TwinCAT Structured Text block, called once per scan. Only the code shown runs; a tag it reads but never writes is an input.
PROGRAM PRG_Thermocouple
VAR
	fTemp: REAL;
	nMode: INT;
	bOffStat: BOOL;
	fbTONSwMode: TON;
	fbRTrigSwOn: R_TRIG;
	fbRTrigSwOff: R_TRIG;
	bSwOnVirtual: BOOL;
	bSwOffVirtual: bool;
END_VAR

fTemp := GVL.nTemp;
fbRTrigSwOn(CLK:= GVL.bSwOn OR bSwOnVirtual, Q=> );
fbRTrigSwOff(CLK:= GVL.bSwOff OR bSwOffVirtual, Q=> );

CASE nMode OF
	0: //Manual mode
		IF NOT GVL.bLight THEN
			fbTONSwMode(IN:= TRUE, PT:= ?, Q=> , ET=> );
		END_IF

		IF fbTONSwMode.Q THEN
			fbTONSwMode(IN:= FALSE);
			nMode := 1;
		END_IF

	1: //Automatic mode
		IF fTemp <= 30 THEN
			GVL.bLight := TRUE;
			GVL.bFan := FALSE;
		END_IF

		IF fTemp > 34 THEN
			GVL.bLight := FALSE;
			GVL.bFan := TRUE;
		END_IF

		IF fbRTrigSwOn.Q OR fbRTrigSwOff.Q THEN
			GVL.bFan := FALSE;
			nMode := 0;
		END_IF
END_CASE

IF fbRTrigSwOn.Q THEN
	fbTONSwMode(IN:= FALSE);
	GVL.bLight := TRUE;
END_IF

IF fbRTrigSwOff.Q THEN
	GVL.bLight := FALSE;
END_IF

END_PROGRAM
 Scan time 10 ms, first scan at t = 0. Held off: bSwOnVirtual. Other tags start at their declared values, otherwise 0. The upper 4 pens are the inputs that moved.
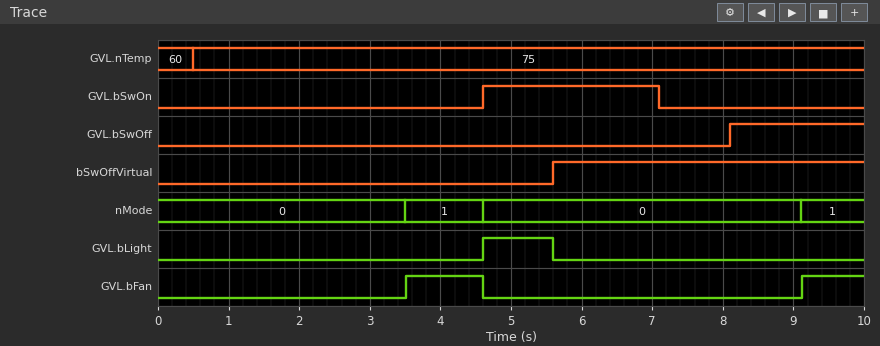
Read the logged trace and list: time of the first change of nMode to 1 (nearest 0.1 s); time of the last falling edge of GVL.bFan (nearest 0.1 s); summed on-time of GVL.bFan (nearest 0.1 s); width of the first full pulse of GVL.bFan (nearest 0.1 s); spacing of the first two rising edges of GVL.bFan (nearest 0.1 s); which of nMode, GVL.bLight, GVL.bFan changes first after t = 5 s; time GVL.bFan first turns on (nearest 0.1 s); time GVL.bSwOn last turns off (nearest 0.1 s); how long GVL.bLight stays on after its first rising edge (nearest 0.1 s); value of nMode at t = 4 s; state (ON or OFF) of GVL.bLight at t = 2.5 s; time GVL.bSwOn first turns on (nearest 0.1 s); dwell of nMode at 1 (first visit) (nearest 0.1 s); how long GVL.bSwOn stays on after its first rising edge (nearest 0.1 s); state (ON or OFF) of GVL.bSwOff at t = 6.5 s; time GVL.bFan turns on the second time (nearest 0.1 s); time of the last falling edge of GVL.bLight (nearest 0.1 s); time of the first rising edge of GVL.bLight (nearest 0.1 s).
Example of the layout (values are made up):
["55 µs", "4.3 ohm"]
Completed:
["3.5 s", "4.6 s", "2.0 s", "1.1 s", "5.6 s", "GVL.bLight", "3.5 s", "7.1 s", "1.0 s", "1", "OFF", "4.6 s", "1.1 s", "2.5 s", "OFF", "9.1 s", "5.6 s", "4.6 s"]
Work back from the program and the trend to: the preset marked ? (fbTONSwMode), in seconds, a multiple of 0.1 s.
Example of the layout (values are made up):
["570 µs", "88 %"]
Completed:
["3.5 s"]
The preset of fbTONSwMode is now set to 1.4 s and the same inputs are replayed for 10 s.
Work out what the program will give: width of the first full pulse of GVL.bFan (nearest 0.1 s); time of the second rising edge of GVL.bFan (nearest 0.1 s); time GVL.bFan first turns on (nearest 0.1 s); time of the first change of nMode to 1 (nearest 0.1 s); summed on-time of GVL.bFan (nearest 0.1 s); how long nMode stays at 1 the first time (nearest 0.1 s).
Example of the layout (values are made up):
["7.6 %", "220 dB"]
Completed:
["3.2 s", "7.0 s", "1.4 s", "1.4 s", "6.2 s", "3.2 s"]
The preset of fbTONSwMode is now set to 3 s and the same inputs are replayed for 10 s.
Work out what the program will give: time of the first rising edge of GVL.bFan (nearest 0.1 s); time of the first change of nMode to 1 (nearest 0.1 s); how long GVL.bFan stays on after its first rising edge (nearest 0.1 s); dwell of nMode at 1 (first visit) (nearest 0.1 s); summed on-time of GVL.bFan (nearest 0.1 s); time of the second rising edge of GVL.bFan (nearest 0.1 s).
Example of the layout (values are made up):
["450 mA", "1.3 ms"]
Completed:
["3.0 s", "3.0 s", "1.6 s", "1.6 s", "3.0 s", "8.6 s"]
